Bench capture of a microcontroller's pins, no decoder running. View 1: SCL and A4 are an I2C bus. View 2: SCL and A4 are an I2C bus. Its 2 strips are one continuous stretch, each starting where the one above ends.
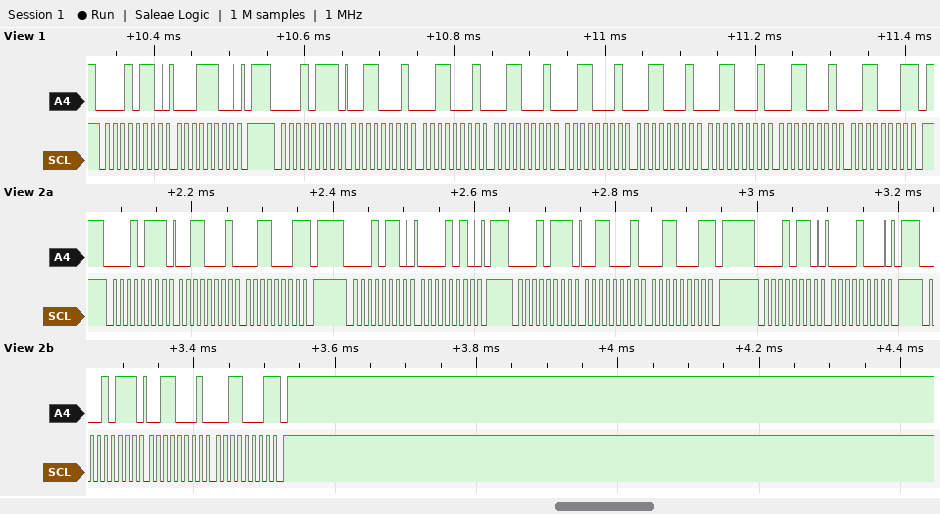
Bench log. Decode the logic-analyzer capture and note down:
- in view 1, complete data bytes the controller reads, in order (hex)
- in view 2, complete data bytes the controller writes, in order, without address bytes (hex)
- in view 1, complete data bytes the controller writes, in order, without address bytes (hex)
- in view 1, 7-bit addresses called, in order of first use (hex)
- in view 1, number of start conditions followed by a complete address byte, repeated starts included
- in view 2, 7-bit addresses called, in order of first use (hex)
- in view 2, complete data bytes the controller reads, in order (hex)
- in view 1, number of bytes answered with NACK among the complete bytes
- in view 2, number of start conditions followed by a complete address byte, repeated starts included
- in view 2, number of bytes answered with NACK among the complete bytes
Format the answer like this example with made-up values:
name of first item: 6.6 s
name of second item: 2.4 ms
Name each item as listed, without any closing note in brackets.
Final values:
in view 1, complete data bytes the controller reads, in order: 31 31 31 31 31 31 31 31
in view 2, complete data bytes the controller writes, in order, without address bytes: 0A 08
in view 1, complete data bytes the controller writes, in order, without address bytes: 1C
in view 1, 7-bit addresses called, in order of first use: 0x0B
in view 1, number of start conditions followed by a complete address byte, repeated starts included: 2
in view 2, 7-bit addresses called, in order of first use: 0x0B
in view 2, complete data bytes the controller reads, in order: 31 31 31 31 31 31
in view 1, number of bytes answered with NACK among the complete bytes: 1
in view 2, number of start conditions followed by a complete address byte, repeated starts included: 5
in view 2, number of bytes answered with NACK among the complete bytes: 3
